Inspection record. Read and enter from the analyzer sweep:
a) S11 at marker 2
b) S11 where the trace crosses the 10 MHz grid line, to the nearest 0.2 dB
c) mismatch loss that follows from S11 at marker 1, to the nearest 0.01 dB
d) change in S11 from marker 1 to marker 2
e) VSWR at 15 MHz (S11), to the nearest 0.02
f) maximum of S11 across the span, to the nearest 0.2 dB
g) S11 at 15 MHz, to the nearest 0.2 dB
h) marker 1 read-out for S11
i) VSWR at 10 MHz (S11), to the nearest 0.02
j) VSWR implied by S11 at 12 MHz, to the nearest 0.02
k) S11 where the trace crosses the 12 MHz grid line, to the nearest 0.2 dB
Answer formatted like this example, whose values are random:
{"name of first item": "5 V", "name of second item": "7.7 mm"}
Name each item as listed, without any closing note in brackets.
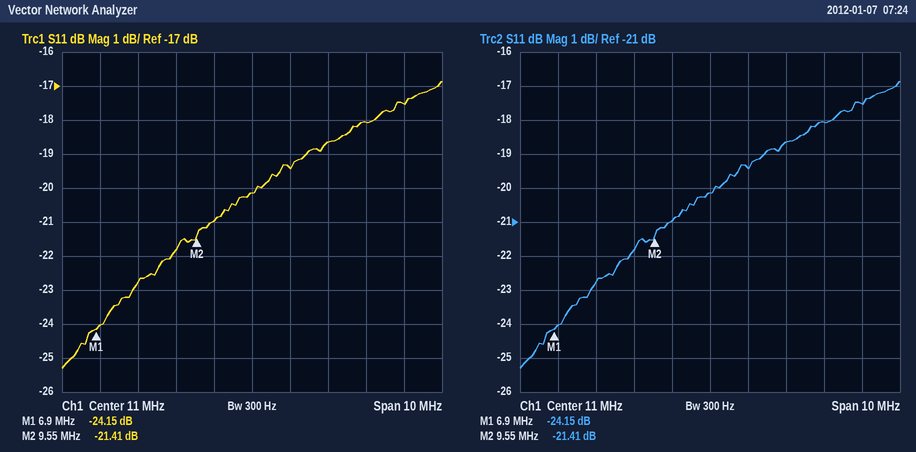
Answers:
{"S11 at marker 2": "-21.41 dB", "S11 where the trace crosses the 10 MHz grid line, to the nearest 0.2 dB": "-21.0 dB", "mismatch loss that follows from S11 at marker 1, to the nearest 0.01 dB": "0.02 dB", "change in S11 from marker 1 to marker 2": "2.74 dB", "VSWR at 15 MHz (S11), to the nearest 0.02": "1.30", "maximum of S11 across the span, to the nearest 0.2 dB": "-16.8 dB", "S11 at 15 MHz, to the nearest 0.2 dB": "-17.6 dB", "marker 1 read-out for S11": "-24.15 dB", "VSWR at 10 MHz (S11), to the nearest 0.02": "1.20", "VSWR implied by S11 at 12 MHz, to the nearest 0.02": "1.24", "S11 where the trace crosses the 12 MHz grid line, to the nearest 0.2 dB": "-19.4 dB"}
